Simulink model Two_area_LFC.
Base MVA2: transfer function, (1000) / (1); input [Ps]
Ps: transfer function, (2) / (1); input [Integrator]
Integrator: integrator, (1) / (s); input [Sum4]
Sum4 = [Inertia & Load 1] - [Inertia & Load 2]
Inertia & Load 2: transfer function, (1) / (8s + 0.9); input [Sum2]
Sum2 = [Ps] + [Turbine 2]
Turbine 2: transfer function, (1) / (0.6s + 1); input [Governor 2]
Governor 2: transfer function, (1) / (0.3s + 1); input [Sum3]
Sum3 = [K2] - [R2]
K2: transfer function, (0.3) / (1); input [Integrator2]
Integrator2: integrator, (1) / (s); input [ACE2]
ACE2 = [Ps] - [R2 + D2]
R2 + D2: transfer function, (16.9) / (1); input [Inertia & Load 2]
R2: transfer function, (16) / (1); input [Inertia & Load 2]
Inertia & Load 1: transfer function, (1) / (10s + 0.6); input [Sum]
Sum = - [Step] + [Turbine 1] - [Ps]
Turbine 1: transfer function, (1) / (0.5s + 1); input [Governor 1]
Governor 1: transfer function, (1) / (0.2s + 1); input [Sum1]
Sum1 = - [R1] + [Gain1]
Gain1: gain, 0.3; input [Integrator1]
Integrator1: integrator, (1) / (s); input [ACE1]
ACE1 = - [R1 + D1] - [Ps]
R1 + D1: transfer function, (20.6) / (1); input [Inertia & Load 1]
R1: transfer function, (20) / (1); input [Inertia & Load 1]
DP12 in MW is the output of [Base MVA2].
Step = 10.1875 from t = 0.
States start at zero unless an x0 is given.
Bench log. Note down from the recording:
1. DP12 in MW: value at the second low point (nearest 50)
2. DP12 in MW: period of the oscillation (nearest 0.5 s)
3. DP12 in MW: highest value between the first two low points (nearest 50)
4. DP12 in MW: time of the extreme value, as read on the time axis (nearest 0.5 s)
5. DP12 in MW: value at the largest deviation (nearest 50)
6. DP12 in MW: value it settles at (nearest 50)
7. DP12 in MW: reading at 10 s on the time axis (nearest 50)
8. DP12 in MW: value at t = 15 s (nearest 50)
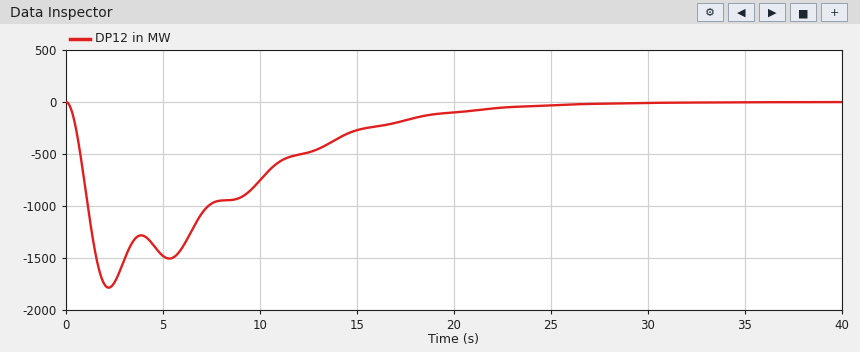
-1500
3.0 s
-1300
2.0 s
-1800
0
-750
-250
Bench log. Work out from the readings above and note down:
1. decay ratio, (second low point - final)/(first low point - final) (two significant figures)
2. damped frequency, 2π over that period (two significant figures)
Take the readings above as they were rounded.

0.83
2.1 rad/s
